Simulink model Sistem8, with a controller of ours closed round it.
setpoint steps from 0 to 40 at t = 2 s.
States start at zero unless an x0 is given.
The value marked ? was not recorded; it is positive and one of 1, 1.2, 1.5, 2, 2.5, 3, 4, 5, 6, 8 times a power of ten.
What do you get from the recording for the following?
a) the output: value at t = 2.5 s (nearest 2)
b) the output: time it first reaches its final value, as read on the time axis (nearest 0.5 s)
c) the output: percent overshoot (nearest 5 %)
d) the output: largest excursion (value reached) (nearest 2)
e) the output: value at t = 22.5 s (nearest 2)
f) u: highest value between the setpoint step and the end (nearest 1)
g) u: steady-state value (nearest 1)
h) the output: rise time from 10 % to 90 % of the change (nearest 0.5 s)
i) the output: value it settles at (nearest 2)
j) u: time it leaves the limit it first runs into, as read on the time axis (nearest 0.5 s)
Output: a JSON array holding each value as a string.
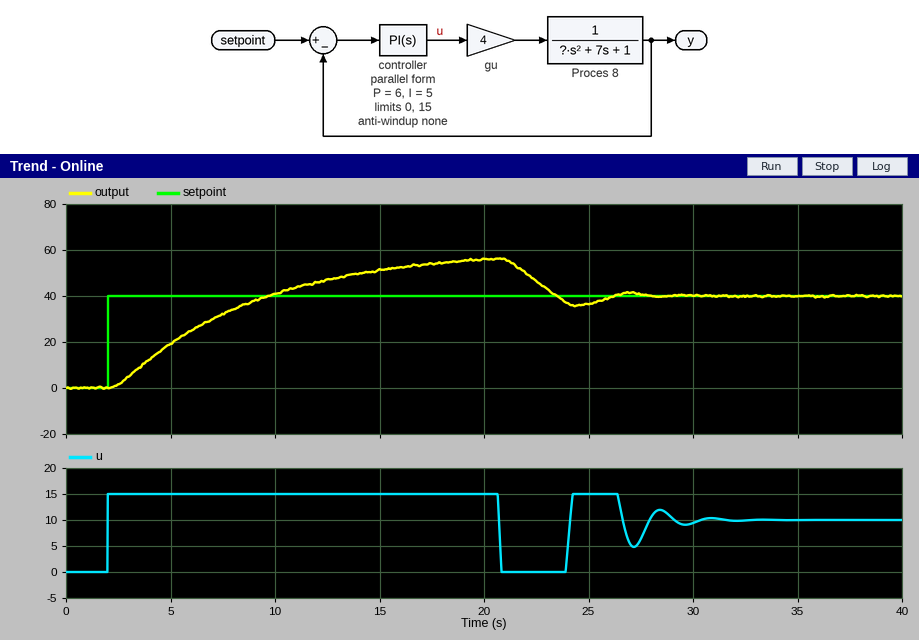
["2", "9.5 s", "40 %", "56", "46", "15", "10", "5.5 s", "40", "20.5 s"]
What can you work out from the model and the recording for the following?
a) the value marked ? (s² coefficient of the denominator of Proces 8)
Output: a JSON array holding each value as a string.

["3"]
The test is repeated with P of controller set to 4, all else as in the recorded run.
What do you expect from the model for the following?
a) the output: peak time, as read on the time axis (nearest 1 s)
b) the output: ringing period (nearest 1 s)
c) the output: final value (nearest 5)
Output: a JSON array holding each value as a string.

["21 s", "9 s", "40"]
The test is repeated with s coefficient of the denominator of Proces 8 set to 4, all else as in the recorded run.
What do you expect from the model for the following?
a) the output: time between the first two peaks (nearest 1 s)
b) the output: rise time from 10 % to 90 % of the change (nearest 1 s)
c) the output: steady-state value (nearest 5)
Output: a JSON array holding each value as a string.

["5 s", "3 s", "40"]
